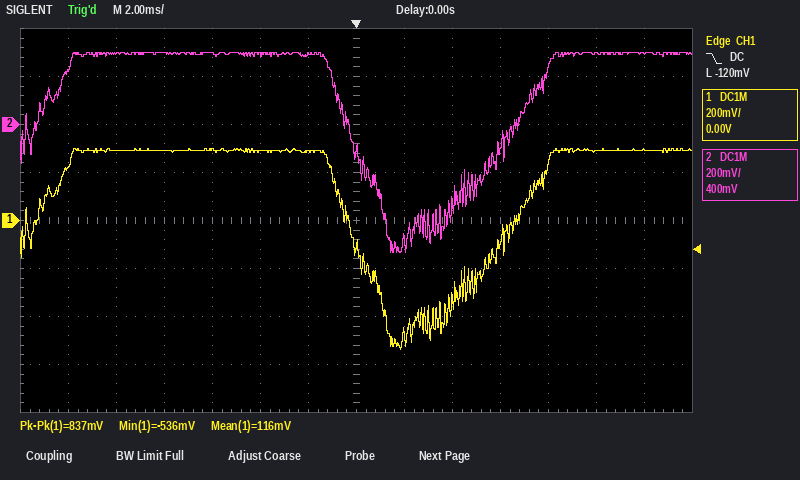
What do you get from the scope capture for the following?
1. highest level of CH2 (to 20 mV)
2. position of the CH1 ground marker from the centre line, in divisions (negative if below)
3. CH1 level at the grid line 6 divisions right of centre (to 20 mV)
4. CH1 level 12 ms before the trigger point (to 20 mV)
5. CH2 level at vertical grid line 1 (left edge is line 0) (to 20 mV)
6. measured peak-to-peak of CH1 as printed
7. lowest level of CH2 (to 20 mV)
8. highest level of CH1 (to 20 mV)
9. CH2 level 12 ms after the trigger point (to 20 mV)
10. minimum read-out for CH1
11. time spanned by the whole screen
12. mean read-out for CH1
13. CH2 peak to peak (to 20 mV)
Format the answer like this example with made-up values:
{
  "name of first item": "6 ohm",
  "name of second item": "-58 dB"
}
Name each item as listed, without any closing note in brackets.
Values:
{
  "highest level of CH2": "300 mV",
  "position of the CH1 ground marker from the centre line, in divisions": "0.0 div",
  "CH1 level at the grid line 6 divisions right of centre": "300 mV",
  "CH1 level 12 ms before the trigger point": "220 mV",
  "CH2 level at vertical grid line 1 (left edge is line 0)": "220 mV",
  "measured peak-to-peak of CH1 as printed": "837 mV",
  "lowest level of CH2": "-540 mV",
  "highest level of CH1": "300 mV",
  "CH2 level 12 ms after the trigger point": "300 mV",
  "minimum read-out for CH1": "-536 mV",
  "time spanned by the whole screen": "28 ms",
  "mean read-out for CH1": "116 mV",
  "CH2 peak to peak": "840 mV"
}
